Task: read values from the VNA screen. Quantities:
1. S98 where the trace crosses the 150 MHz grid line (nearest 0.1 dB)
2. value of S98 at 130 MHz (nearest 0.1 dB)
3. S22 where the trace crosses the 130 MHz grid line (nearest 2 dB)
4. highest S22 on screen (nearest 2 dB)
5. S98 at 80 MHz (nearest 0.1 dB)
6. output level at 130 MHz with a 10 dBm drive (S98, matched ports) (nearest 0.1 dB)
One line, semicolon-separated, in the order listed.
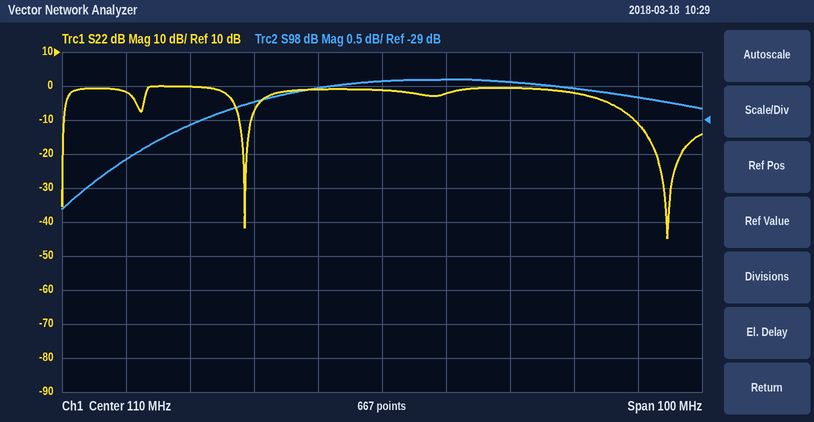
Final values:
-28.7 dB; -28.4 dB; 0 dB; 0 dB; -29.1 dB; -18.4 dBm
